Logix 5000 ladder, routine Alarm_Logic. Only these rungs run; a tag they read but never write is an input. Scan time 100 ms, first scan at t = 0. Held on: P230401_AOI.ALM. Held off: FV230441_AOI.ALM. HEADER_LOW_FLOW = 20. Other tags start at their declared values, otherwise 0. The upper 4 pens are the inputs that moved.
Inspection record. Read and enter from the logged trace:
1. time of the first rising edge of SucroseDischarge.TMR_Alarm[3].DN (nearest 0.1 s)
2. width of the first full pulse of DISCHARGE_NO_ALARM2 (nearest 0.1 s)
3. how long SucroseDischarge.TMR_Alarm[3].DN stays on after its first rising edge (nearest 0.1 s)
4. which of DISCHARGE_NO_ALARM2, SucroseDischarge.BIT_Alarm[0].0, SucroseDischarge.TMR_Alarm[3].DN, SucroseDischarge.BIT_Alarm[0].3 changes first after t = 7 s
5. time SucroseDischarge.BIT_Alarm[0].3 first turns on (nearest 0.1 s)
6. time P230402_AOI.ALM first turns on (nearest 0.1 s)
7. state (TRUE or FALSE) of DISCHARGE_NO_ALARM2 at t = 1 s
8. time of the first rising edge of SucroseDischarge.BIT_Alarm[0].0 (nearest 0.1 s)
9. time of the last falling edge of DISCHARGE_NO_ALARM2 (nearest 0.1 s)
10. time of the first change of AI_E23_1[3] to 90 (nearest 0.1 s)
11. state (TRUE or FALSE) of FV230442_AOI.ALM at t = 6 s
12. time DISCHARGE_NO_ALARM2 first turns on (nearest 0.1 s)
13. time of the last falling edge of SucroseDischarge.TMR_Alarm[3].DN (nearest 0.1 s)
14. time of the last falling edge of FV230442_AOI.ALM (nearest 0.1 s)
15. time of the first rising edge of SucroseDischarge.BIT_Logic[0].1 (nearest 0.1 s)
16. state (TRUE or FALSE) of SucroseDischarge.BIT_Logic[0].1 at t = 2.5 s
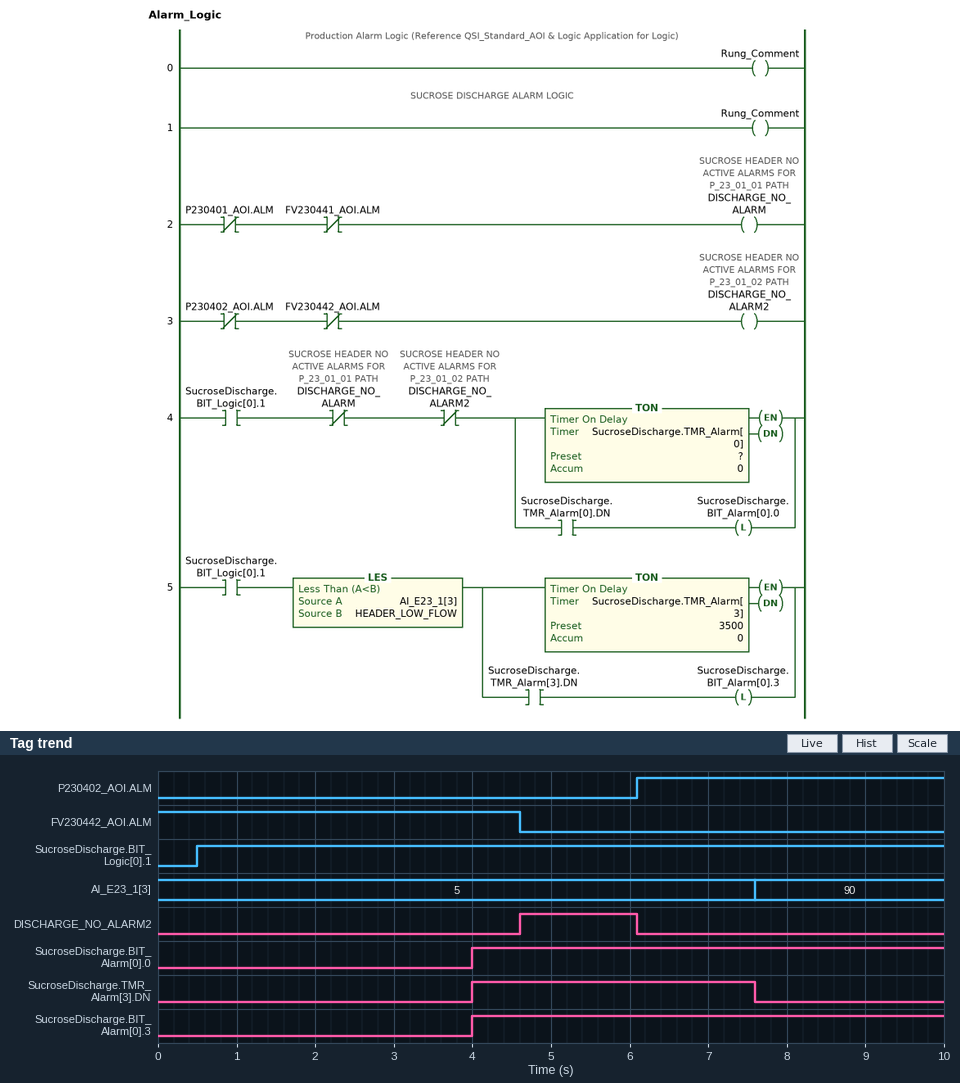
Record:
4.0 s
1.5 s
3.6 s
SucroseDischarge.TMR_Alarm[3].DN
4.0 s
6.1 s
FALSE
4.0 s
6.1 s
7.6 s
FALSE
4.6 s
7.6 s
4.6 s
0.5 s
TRUE
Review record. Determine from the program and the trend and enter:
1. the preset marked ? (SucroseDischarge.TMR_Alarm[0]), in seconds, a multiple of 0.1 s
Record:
3.5 s
